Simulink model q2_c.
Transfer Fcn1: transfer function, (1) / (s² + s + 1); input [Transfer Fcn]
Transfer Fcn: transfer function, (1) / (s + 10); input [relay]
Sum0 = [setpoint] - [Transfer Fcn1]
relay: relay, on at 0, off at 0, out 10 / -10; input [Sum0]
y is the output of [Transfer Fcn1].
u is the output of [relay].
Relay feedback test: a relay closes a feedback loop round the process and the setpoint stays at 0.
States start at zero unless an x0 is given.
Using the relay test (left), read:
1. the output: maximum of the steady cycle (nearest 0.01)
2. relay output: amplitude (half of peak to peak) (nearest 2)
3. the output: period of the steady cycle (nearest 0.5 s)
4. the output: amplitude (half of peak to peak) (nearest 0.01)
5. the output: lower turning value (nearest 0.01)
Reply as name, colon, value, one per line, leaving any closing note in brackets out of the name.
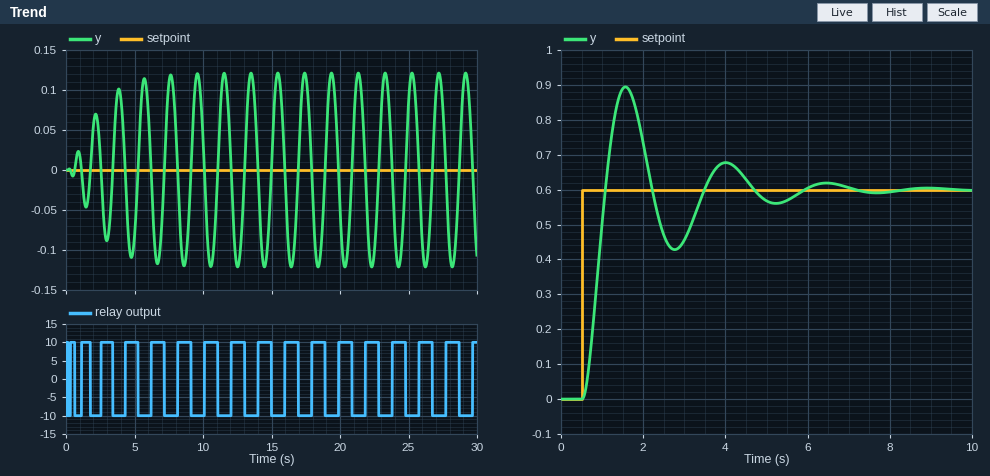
the output: maximum of the steady cycle: 0.12
relay output: amplitude (half of peak to peak): 10
the output: period of the steady cycle: 2.0 s
the output: amplitude (half of peak to peak): 0.12
the output: lower turning value: -0.12
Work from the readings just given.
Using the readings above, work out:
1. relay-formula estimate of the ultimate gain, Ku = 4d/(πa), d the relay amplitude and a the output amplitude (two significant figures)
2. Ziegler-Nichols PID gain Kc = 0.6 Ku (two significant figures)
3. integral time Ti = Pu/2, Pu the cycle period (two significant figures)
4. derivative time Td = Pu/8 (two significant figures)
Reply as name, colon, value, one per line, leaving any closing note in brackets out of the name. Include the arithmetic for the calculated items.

relay-formula estimate of the ultimate gain, Ku = 4d/(πa), d the relay amplitude and a the output amplitude: 4 × 10 / (π × 0.12) = 110
Ziegler-Nichols PID gain Kc = 0.6 Ku: 0.6 × 110 = 66
integral time Ti = Pu/2, Pu the cycle period: 2 / 2 = 1.0 s
derivative time Td = Pu/8: 2 / 8 = 0.25 s
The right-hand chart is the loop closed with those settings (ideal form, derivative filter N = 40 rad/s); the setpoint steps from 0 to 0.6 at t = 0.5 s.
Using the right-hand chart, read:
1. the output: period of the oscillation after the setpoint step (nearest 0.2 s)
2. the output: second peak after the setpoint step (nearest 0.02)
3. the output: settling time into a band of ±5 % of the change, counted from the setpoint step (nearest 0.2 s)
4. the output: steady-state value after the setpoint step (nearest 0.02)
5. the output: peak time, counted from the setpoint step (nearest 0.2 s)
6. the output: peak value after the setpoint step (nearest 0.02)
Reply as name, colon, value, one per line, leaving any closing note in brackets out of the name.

the output: period of the oscillation after the setpoint step: 2.4 s
the output: second peak after the setpoint step: 0.68
the output: settling time into a band of ±5 % of the change, counted from the setpoint step: 5.0 s
the output: steady-state value after the setpoint step: 0.60
the output: peak time, counted from the setpoint step: 1.0 s
the output: peak value after the setpoint step: 0.90
